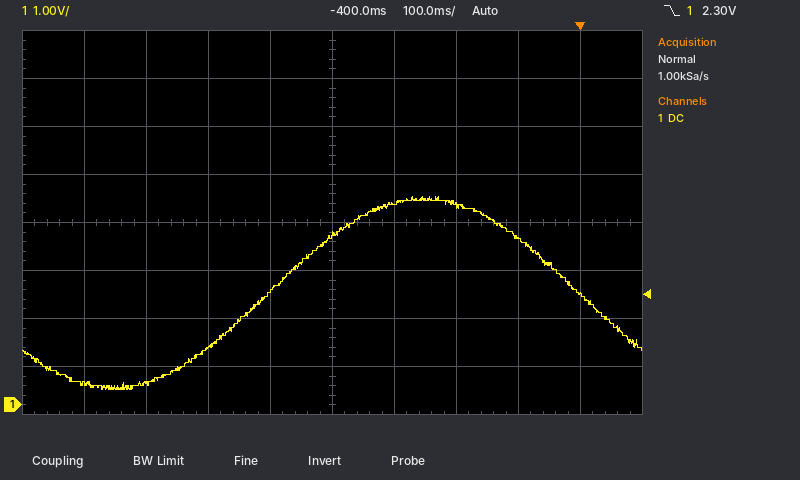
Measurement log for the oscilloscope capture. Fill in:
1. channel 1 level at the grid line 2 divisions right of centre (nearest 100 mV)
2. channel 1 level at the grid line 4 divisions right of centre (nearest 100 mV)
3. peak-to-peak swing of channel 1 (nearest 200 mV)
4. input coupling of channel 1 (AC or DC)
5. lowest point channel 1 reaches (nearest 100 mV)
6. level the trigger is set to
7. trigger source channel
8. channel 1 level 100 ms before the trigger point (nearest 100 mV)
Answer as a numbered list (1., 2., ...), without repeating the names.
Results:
1. 4.2 V
2. 2.3 V
3. 4.0 V
4. DC
5. 300 mV
6. 2.30 V
7. channel 1
8. 3.5 V
